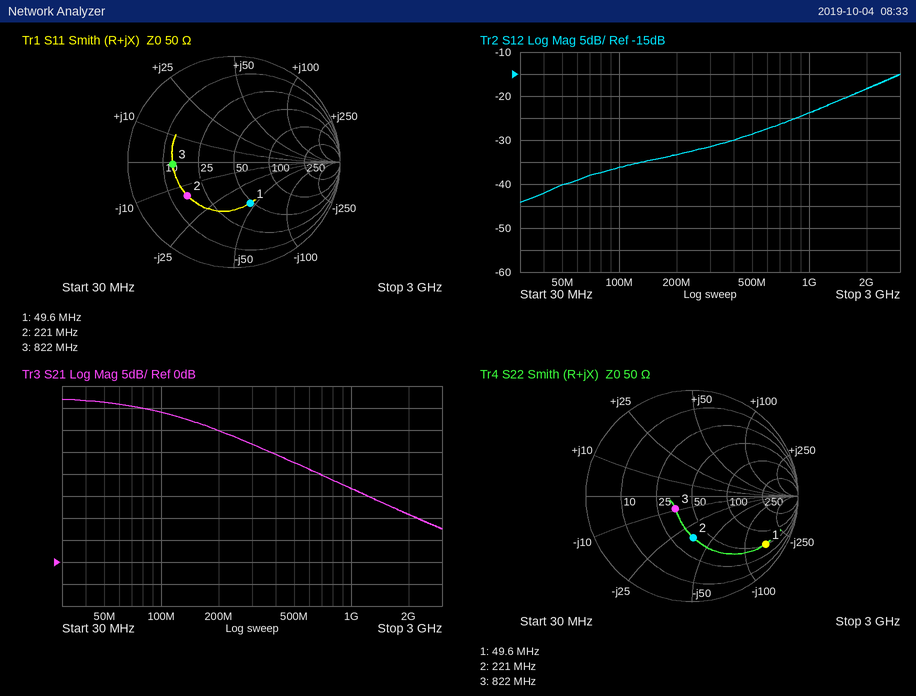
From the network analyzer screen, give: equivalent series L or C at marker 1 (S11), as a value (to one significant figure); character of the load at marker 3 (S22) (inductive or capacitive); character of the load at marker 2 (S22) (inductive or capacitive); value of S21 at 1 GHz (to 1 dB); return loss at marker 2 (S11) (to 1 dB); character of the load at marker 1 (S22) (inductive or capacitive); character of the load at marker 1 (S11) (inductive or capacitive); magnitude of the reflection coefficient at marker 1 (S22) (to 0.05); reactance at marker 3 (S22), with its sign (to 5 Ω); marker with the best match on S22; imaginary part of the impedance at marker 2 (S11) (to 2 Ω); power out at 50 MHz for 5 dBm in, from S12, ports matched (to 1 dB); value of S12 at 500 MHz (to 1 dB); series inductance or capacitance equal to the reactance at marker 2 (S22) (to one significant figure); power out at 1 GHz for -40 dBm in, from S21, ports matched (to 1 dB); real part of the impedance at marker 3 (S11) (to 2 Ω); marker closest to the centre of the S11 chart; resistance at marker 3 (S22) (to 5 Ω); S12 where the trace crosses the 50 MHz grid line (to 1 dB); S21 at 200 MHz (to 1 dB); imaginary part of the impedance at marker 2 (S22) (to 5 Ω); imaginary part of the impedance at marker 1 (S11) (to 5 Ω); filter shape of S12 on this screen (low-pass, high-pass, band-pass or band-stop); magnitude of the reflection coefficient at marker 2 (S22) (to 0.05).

70 pF
capacitive
capacitive
17 dB
5 dB
capacitive
capacitive
0.85
-10 Ω
marker 3
-14 Ω
-35 dBm
-29 dB
20 pF
-23 dBm
14 Ω
marker 1
35 Ω
-40 dB
30 dB
-35 Ω
-45 Ω
high-pass
0.40
